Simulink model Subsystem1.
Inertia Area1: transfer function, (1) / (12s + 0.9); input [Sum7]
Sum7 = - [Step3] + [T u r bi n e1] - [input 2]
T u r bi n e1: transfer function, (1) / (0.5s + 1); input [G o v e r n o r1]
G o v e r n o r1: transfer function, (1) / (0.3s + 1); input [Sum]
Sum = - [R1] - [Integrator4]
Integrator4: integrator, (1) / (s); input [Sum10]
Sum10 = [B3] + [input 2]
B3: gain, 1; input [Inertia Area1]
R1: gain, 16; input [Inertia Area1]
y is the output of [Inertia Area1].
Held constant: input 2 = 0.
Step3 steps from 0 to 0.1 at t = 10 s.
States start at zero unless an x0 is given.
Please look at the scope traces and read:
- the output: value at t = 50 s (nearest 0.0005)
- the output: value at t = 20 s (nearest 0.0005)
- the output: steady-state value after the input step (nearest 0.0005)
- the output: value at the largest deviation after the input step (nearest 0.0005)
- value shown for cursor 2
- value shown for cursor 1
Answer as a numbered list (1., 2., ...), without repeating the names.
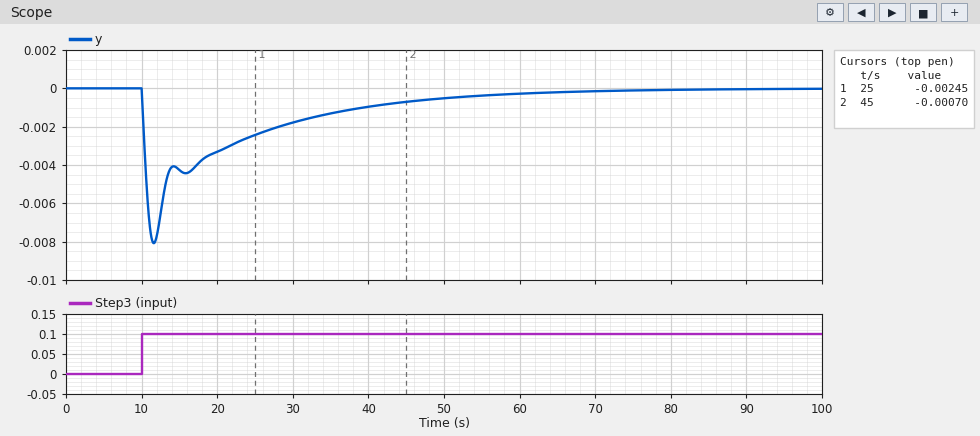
1. -0.0005
2. -0.0035
3. 0.0000
4. -0.0080
5. -0.00070
6. -0.00245
